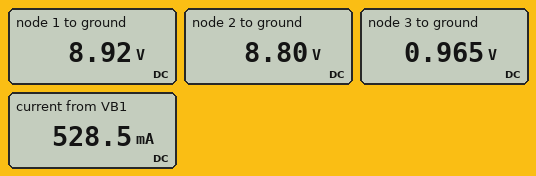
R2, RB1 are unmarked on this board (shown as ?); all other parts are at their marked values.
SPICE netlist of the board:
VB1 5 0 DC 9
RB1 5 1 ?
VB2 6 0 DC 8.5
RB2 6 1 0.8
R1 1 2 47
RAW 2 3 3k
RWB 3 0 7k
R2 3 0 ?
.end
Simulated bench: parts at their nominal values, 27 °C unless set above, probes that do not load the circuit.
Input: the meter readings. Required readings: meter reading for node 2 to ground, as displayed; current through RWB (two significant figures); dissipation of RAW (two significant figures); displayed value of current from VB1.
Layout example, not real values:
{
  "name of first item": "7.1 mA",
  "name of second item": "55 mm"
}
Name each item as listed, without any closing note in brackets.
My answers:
{
  "meter reading for node 2 to ground, as displayed": "8.80 V",
  "current through RWB": "140 µA",
  "dissipation of RAW": "20 mW",
  "displayed value of current from VB1": "528.5 mA"
}
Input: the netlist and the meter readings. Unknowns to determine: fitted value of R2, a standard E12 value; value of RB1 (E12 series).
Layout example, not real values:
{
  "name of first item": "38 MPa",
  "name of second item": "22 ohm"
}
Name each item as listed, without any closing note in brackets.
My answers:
{
  "fitted value of R2, a standard E12 value": "390 Ω",
  "value of RB1": "0.15 Ω"
}
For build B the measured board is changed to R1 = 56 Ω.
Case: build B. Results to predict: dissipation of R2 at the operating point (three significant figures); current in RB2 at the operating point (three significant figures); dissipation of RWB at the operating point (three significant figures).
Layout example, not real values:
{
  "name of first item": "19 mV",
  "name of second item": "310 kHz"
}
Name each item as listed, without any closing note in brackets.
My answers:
{
  "dissipation of R2 at the operating point": "2.37 mW",
  "current in RB2 at the operating point": "526 mA",
  "dissipation of RWB at the operating point": "132 µW"
}
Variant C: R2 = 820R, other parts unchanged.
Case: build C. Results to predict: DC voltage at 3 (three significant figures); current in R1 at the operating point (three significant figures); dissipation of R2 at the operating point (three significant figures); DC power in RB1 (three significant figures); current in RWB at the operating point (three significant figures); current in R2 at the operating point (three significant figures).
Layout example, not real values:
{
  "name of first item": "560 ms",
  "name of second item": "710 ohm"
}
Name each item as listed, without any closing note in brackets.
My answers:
{
  "DC voltage at 3": "1.73 V",
  "current in R1 at the operating point": "2.36 mA",
  "dissipation of R2 at the operating point": "3.66 mW",
  "DC power in RB1": "41.9 mW",
  "current in RWB at the operating point": "247 µA",
  "current in R2 at the operating point": "2.11 mA"
}
